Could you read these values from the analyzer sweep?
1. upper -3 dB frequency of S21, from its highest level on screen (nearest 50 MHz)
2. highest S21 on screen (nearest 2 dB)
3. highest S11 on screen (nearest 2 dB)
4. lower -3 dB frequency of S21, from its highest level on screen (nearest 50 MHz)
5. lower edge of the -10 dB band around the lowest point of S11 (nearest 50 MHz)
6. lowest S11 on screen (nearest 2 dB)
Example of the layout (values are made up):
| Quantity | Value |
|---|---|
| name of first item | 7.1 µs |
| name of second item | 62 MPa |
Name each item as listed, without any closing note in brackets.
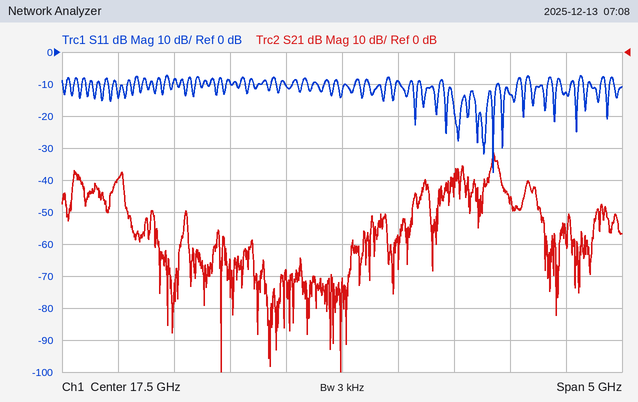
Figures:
| Quantity | Value |
|---|---|
| upper -3 dB frequency of S21, from its highest level on screen | 18.90 GHz |
| highest S21 on screen | -32 dB |
| highest S11 on screen | -8 dB |
| lower -3 dB frequency of S21, from its highest level on screen | 18.85 GHz |
| lower edge of the -10 dB band around the lowest point of S11 | 18.40 GHz |
| lowest S11 on screen | -38 dB |
